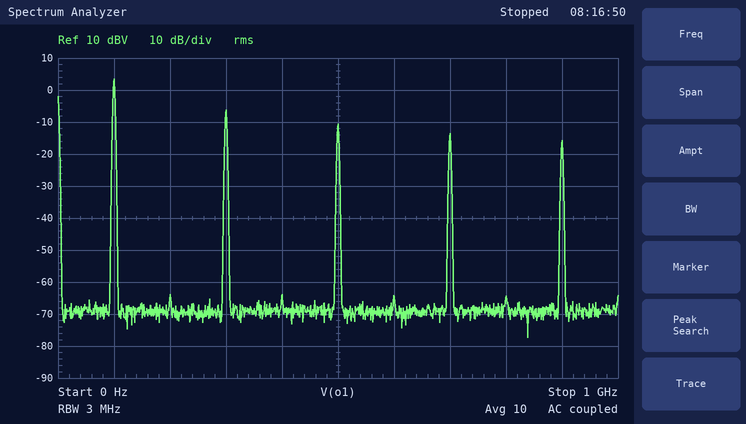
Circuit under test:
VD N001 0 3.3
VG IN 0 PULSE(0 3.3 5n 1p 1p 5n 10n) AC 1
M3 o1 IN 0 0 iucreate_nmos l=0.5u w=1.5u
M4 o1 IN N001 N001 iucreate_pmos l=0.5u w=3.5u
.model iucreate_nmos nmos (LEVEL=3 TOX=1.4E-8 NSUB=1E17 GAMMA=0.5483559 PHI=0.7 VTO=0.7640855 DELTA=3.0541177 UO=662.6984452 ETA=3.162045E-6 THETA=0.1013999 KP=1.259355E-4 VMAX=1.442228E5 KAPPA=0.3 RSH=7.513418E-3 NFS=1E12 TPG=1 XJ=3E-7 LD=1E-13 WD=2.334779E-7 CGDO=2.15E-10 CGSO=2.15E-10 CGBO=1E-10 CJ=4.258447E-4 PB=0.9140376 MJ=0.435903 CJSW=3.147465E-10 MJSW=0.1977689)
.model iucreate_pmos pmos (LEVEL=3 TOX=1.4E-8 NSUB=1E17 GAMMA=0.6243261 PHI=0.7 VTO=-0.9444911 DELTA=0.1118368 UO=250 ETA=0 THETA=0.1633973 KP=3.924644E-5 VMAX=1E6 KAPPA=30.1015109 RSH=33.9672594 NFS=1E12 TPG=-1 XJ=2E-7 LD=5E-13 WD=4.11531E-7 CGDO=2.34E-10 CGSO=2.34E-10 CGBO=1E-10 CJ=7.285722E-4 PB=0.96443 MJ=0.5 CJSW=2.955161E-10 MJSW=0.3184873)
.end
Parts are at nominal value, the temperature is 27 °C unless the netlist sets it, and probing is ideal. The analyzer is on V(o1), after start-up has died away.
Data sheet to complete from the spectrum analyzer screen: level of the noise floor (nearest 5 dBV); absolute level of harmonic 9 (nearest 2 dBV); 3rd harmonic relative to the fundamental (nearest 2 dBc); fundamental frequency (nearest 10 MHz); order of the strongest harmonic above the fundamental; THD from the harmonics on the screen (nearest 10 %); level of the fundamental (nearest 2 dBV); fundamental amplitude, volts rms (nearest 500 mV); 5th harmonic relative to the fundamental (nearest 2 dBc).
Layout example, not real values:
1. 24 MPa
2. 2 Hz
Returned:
1. -70 dBV
2. -16 dBV
3. -10 dBc
4. 100 MHz
5. 3
6. 40 %
7. 4 dBV
8. 1.5 V
9. -14 dBc
